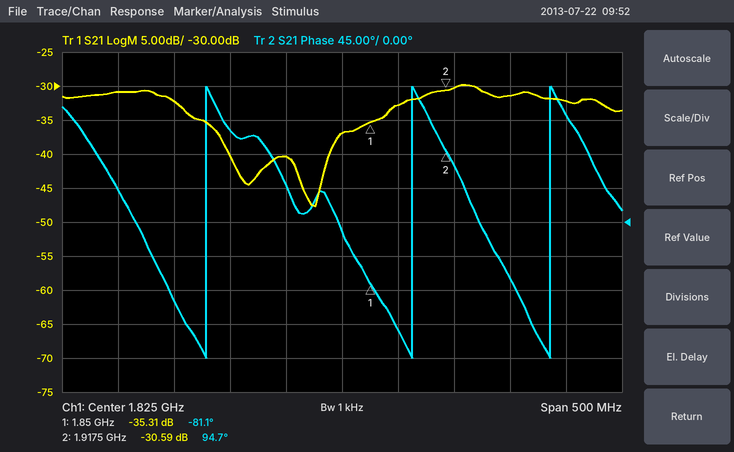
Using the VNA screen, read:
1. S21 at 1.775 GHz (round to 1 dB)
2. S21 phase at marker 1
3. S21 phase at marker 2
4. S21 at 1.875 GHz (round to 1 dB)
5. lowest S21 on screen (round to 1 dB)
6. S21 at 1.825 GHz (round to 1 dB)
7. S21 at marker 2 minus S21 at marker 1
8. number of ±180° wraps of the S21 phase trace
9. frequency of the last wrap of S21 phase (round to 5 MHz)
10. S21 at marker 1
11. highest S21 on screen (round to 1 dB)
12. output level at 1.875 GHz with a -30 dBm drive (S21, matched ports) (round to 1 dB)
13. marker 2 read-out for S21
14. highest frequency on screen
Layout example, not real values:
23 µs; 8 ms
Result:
-40 dB; -81.1°; 94.7°; -33 dB; -48 dB; -37 dB; 4.72 dB; 3; 2.010 GHz; -35.31 dB; -30 dB; -63 dBm; -30.59 dB; 2.075 GHz
